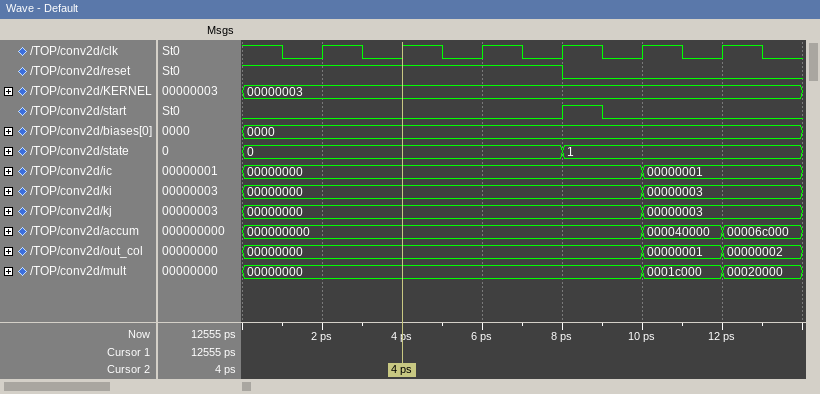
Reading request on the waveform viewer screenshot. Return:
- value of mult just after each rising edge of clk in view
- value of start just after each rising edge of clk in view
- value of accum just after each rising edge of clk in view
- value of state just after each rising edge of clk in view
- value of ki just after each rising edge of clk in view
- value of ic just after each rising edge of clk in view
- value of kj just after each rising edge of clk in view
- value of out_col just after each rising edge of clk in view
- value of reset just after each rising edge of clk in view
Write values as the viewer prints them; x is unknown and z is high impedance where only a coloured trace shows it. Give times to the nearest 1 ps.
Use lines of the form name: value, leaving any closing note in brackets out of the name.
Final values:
value of mult just after each rising edge of clk in view: 00000000, 00000000, 00000000, 00000000, 0001c000, 00020000
value of start just after each rising edge of clk in view: 0 0 0 1 0 0
value of accum just after each rising edge of clk in view: 000000000, 000000000, 000000000, 000000000, 000040000, 00006c000
value of state just after each rising edge of clk in view: 0, 0, 0, 1, 1, 1
value of ki just after each rising edge of clk in view: 00000000, 00000000, 00000000, 00000000, 00000003, 00000003
value of ic just after each rising edge of clk in view: 00000000, 00000000, 00000000, 00000000, 00000001, 00000001
value of kj just after each rising edge of clk in view: 00000000, 00000000, 00000000, 00000000, 00000003, 00000003
value of out_col just after each rising edge of clk in view: 00000000, 00000000, 00000000, 00000000, 00000001, 00000002
value of reset just after each rising edge of clk in view: 1 1 1 0 0 0
